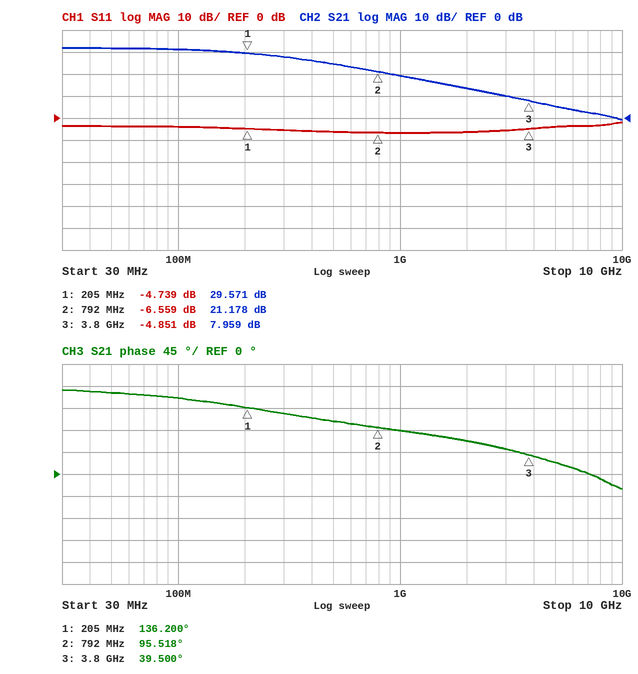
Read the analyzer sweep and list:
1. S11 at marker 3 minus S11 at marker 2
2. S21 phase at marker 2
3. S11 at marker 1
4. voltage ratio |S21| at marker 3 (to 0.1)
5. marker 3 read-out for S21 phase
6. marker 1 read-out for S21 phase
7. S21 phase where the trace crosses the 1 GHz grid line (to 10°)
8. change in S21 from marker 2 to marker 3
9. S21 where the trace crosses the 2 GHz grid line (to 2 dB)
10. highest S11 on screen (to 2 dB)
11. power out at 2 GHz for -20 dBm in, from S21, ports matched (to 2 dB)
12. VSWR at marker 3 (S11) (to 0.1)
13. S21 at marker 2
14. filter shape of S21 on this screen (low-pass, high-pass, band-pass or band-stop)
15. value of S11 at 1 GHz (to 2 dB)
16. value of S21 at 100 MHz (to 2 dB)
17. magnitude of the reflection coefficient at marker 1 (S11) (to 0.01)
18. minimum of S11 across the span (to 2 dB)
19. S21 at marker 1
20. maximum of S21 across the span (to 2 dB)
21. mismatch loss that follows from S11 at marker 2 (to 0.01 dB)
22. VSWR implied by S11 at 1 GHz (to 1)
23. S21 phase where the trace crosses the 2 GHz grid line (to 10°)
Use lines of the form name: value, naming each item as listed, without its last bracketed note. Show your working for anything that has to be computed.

S11 at marker 3 minus S11 at marker 2: -4.851 − (-6.559) = 1.708 dB
S21 phase at marker 2: 95.518°
S11 at marker 1: -4.739 dB
voltage ratio |S21| at marker 3: 10^(7.959/20) ≈ 2.5
marker 3 read-out for S21 phase: 39.500°
marker 1 read-out for S21 phase: 136.200°
S21 phase where the trace crosses the 1 GHz grid line: 90°
change in S21 from marker 2 to marker 3: 7.959 − (21.178) = -13.219 dB
S21 where the trace crosses the 2 GHz grid line: 14 dB
highest S11 on screen: -2 dB
power out at 2 GHz for -20 dBm in, from S21, ports matched: -20 dBm + (14 dB) = -6 dBm
VSWR at marker 3 (S11): (1 + 0.5721)/(1 − 0.5721) ≈ 3.7
S21 at marker 2: 21.178 dB
filter shape of S21 on this screen: low-pass
value of S11 at 1 GHz: -6 dB
value of S21 at 100 MHz: 32 dB
magnitude of the reflection coefficient at marker 1 (S11): 10^(-4.739/20) ≈ 0.58
minimum of S11 across the span: -6 dB
S21 at marker 1: 29.571 dB
maximum of S21 across the span: 32 dB
mismatch loss that follows from S11 at marker 2: −10 log10(1 − 10^(-6.559/10)) ≈ 1.08 dB
VSWR implied by S11 at 1 GHz: |Γ| = 10^(-6/20) = 0.5012; VSWR = (1 + 0.5012)/(1 − 0.5012) ≈ 3
S21 phase where the trace crosses the 2 GHz grid line: 70°
